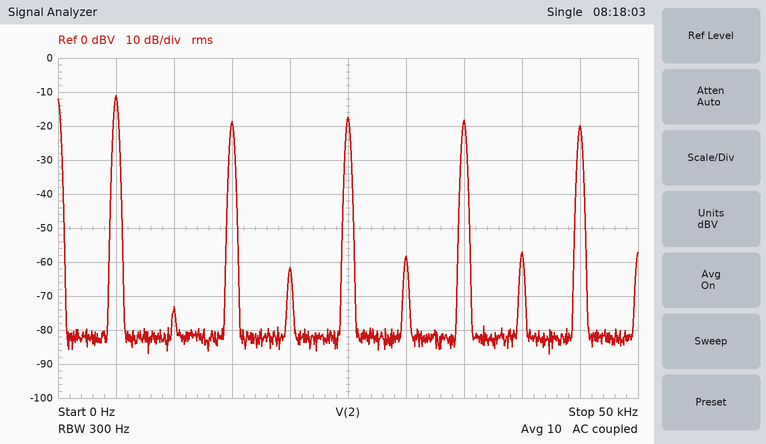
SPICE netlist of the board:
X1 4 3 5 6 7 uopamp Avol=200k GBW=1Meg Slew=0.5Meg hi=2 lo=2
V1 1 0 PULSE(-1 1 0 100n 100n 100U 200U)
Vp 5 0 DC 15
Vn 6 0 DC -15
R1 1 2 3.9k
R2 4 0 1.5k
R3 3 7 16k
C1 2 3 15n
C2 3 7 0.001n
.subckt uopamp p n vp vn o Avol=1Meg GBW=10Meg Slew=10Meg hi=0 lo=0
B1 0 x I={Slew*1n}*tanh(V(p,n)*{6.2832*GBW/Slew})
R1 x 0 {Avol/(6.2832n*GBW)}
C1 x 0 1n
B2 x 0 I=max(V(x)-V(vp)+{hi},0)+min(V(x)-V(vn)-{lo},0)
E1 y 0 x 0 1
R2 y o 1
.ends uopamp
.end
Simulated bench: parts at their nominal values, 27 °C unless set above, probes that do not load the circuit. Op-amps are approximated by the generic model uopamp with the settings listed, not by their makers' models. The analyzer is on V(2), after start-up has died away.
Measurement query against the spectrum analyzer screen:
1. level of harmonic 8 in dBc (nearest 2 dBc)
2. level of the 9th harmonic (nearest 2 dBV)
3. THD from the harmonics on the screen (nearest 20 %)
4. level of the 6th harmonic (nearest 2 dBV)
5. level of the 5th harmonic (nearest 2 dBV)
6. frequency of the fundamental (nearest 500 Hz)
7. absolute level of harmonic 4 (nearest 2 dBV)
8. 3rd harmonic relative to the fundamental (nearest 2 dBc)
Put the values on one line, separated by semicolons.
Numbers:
-46 dBc; -20 dBV; 80 %; -58 dBV; -18 dBV; 5.0 kHz; -62 dBV; -8 dBc
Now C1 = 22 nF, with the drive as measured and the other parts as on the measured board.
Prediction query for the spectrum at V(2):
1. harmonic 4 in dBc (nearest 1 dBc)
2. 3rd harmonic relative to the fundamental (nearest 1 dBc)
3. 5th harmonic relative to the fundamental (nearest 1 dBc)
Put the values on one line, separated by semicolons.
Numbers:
-44 dBc; -1 dBc; 0 dBc
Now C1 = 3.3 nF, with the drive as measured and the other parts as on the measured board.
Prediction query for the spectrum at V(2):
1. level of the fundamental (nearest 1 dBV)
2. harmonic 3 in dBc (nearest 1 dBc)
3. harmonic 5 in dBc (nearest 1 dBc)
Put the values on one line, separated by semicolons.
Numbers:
-2 dBV; -18 dBc; -23 dBc
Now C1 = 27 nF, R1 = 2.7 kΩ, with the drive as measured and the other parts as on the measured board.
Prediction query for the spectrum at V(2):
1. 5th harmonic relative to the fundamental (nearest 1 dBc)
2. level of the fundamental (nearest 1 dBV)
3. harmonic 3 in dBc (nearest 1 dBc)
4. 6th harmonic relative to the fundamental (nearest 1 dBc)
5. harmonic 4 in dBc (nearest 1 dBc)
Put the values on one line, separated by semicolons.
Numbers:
3 dBc; -18 dBV; 4 dBc; -39 dBc; -40 dBc
